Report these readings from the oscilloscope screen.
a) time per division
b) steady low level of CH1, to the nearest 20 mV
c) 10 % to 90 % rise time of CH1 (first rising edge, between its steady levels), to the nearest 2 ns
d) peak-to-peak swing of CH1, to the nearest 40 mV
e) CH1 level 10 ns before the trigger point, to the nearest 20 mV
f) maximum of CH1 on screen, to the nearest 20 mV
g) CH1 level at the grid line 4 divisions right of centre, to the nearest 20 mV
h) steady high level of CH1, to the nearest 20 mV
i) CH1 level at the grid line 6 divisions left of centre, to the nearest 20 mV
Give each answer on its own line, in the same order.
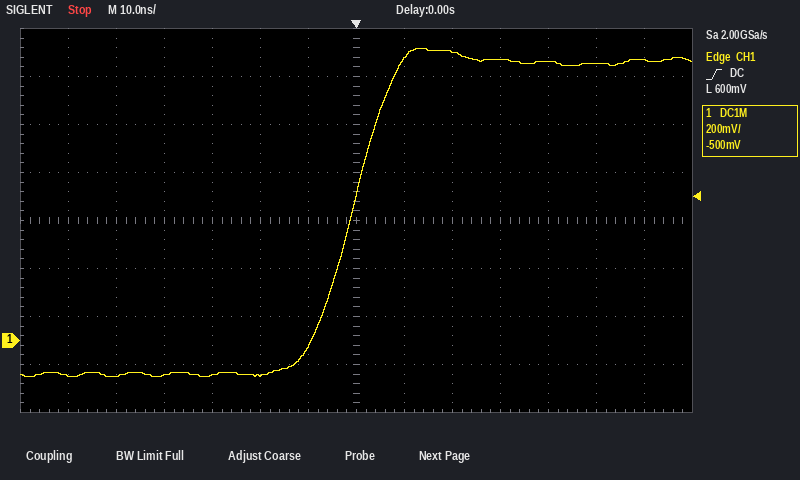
10 ns
-140 mV
16 ns
1.36 V
-20 mV
1.22 V
1.16 V
1.16 V
-140 mV
